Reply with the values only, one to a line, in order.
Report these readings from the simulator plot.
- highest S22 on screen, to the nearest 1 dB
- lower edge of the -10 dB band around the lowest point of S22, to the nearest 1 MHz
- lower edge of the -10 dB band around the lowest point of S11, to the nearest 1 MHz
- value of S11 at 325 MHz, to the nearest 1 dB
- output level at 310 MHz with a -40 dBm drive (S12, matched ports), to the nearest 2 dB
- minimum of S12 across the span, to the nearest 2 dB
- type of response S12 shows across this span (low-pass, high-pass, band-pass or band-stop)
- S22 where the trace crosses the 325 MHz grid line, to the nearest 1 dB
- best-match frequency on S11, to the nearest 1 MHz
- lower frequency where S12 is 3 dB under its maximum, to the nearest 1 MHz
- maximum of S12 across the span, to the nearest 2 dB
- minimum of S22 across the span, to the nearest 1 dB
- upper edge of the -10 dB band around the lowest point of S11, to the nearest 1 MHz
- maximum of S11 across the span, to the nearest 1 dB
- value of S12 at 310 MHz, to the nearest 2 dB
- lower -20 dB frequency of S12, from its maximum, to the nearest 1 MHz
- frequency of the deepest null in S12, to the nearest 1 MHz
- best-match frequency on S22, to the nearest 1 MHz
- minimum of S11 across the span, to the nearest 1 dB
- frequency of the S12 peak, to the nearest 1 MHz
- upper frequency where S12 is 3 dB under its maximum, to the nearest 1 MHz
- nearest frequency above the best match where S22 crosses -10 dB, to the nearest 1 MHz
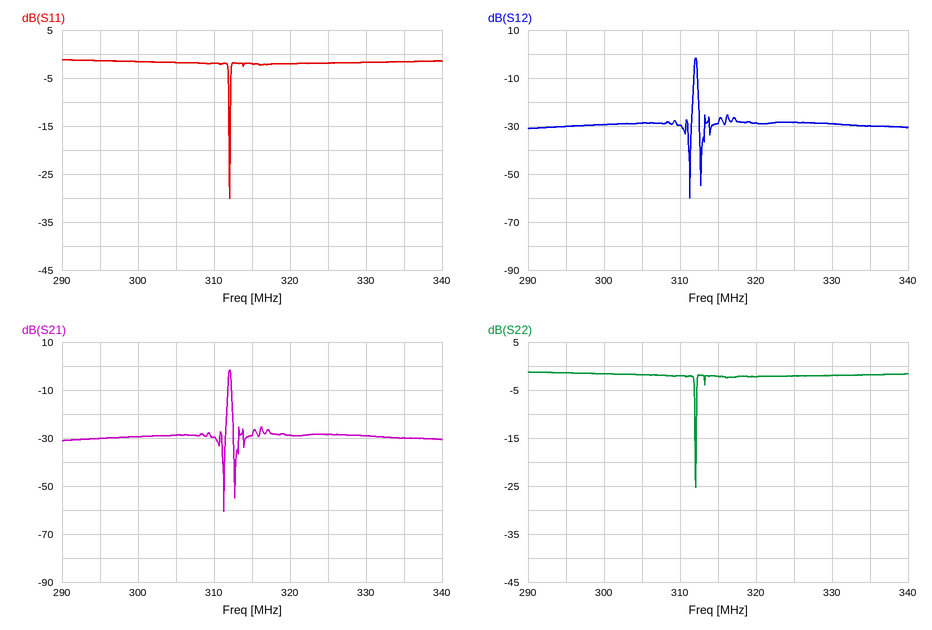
-1 dB
312 MHz
312 MHz
-2 dB
-70 dBm
-60 dB
band-pass
-2 dB
312 MHz
312 MHz
-2 dB
-25 dB
312 MHz
-1 dB
-30 dB
312 MHz
311 MHz
312 MHz
-30 dB
312 MHz
312 MHz
312 MHz
